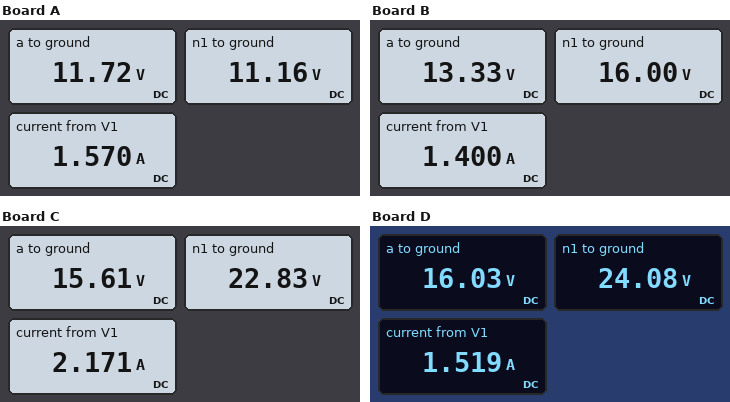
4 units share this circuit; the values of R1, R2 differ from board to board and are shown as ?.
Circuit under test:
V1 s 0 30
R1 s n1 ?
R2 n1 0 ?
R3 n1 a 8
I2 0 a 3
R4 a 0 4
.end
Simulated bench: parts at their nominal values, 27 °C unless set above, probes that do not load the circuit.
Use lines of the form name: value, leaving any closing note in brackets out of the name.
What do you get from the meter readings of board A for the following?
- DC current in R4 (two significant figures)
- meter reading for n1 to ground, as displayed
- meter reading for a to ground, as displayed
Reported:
DC current in R4: 2.9 A
meter reading for n1 to ground, as displayed: 11.16 V
meter reading for a to ground, as displayed: 11.72 V
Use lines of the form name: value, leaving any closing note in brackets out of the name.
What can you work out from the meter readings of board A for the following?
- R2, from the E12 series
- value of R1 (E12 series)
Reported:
R2, from the E12 series: 6.8 Ω
value of R1: 12 Ω
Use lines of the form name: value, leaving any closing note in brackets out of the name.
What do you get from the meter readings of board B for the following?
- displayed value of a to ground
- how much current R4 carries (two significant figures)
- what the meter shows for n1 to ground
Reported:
displayed value of a to ground: 13.33 V
how much current R4 carries: 3.3 A
what the meter shows for n1 to ground: 16.00 V
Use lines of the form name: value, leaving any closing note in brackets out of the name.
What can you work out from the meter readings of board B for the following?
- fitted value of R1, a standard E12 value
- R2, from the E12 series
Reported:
fitted value of R1, a standard E12 value: 10 Ω
R2, from the E12 series: 15 Ω
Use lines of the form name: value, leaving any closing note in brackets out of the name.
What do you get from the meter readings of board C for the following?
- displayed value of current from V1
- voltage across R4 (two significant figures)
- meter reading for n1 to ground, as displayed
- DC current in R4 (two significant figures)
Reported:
displayed value of current from V1: 2.171 A
voltage across R4: 16 V
meter reading for n1 to ground, as displayed: 22.83 V
DC current in R4: 3.9 A
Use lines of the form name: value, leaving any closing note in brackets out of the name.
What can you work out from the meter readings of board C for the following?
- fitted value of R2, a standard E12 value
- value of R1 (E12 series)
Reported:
fitted value of R2, a standard E12 value: 18 Ω
value of R1: 3.3 Ω
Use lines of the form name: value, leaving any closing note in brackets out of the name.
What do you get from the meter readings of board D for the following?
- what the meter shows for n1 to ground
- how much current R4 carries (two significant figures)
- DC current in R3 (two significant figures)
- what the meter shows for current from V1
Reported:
what the meter shows for n1 to ground: 24.08 V
how much current R4 carries: 4.0 A
DC current in R3: 1.0 A
what the meter shows for current from V1: 1.519 A
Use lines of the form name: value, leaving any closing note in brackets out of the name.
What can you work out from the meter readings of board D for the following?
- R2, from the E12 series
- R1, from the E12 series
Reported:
R2, from the E12 series: 47 Ω
R1, from the E12 series: 3.9 Ω
